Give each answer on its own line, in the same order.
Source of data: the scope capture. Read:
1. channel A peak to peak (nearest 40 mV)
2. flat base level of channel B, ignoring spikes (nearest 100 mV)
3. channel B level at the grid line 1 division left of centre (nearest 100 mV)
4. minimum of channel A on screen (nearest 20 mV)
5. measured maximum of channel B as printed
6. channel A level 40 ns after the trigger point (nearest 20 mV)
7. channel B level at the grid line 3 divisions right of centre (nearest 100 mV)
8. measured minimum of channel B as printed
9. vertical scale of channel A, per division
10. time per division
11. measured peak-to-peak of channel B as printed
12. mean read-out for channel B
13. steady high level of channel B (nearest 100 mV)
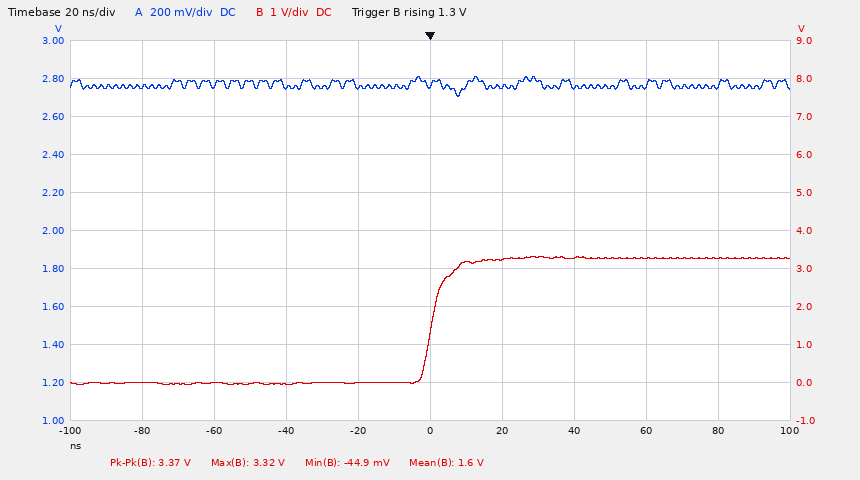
120 mV
0.0 V
0.0 V
2.70 V
3.32 V
2.76 V
3.3 V
-44.9 mV
200 mV
20 ns
3.37 V
1.6 V
3.3 V
